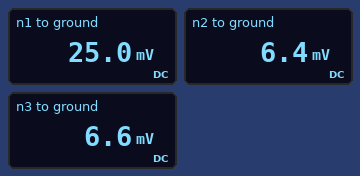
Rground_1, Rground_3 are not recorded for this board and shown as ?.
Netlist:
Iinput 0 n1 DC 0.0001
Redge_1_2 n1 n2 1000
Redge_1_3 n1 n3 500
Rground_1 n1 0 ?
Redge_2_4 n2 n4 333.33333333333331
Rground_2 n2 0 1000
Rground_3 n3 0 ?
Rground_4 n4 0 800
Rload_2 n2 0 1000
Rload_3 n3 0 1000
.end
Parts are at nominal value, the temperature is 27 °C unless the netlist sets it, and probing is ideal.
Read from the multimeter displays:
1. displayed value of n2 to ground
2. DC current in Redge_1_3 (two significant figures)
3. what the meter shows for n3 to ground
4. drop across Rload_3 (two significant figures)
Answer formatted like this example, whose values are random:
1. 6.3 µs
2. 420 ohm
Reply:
1. 6.4 mV
2. 37 µA
3. 6.6 mV
4. 6.6 mV
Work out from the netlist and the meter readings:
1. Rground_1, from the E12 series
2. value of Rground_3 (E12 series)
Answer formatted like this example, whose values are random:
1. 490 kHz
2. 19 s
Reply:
1. 560 Ω
2. 220 Ω
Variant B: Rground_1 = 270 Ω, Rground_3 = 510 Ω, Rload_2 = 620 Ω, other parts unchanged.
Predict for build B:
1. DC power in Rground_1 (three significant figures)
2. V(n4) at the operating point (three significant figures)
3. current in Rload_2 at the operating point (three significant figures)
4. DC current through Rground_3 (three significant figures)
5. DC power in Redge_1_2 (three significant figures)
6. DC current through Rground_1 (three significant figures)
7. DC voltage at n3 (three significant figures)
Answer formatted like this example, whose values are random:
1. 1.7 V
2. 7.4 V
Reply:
1. 1.15 µW
2. 2.77 mV
3. 6.32 µA
4. 13.9 µA
5. 188 nW
6. 65.3 µA
7. 7.10 mV
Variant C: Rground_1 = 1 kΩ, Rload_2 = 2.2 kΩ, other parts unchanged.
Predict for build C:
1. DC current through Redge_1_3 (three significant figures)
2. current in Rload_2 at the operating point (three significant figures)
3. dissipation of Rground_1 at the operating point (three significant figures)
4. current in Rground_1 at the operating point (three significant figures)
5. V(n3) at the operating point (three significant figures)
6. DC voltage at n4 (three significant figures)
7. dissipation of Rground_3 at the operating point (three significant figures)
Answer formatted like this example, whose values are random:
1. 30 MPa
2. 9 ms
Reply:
1. 46.4 µA
2. 4.30 µA
3. 995 nW
4. 31.5 µA
5. 8.36 mV
6. 6.67 mV
7. 318 nW
